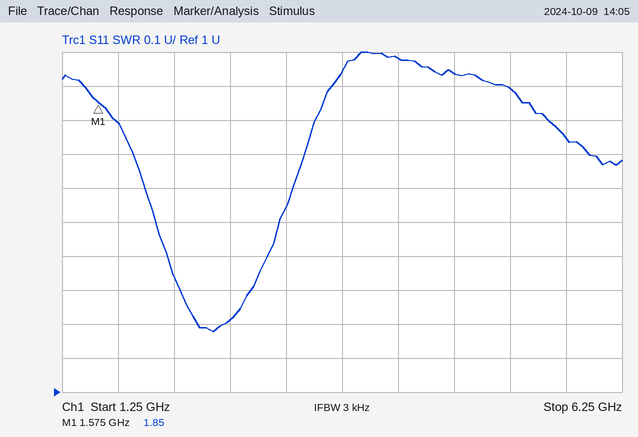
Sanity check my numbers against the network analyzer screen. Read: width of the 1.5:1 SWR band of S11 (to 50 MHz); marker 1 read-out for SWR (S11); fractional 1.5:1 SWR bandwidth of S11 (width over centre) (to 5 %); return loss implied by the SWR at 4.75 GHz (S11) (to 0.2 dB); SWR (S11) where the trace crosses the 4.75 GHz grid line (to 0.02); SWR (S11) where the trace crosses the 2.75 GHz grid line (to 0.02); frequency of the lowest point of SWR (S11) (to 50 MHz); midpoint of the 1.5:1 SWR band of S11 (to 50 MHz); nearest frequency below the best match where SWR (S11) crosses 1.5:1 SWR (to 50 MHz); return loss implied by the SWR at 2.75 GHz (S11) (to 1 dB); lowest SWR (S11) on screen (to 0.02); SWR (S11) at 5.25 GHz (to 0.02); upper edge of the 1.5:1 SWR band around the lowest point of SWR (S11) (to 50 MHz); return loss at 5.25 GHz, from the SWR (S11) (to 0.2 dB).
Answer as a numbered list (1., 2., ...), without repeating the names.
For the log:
1. 1.10 GHz
2. 1.85
3. 40 %
4. 10.0 dB
5. 1.94
6. 1.22
7. 2.60 GHz
8. 2.65 GHz
9. 2.10 GHz
10. 20 dB
11. 1.18
12. 1.90
13. 3.20 GHz
14. 10.2 dB
